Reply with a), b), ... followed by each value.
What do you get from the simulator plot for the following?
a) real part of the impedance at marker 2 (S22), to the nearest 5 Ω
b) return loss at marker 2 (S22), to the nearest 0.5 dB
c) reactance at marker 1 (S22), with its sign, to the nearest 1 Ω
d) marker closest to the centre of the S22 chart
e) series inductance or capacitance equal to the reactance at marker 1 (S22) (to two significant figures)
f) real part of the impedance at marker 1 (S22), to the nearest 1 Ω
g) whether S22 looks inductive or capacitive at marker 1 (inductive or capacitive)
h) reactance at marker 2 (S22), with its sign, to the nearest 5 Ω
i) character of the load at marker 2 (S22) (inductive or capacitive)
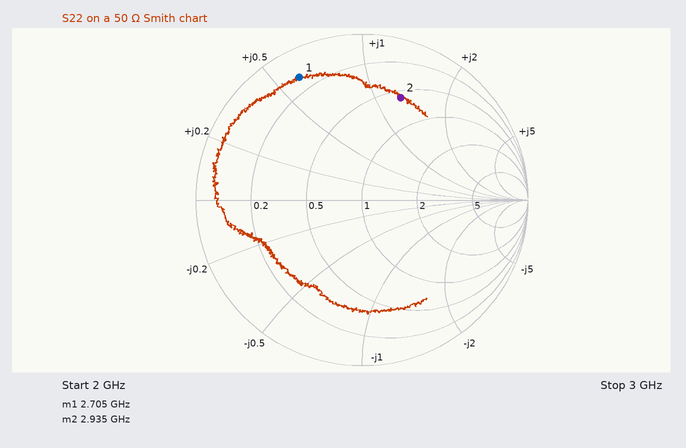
a) 30 Ω
b) 3.5 dB
c) +30 Ω
d) marker 2
e) 1.8 nH
f) 6 Ω
g) inductive
h) +65 Ω
i) inductive
